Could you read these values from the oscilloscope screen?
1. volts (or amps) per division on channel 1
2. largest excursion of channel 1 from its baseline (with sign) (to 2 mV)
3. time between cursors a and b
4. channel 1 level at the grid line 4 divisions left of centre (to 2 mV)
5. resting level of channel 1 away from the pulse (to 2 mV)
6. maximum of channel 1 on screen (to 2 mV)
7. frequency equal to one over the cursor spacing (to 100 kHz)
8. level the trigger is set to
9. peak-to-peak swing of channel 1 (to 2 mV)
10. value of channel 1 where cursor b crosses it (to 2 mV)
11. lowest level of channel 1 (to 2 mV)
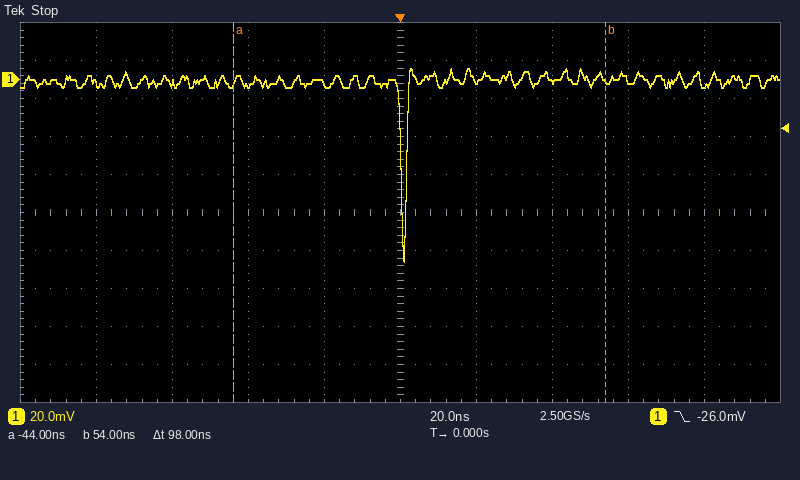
20 mV
-96 mV
98 ns
-2 mV
0 mV
6 mV
10.2 MHz
-26.0 mV
102 mV
0 mV
-96 mV
